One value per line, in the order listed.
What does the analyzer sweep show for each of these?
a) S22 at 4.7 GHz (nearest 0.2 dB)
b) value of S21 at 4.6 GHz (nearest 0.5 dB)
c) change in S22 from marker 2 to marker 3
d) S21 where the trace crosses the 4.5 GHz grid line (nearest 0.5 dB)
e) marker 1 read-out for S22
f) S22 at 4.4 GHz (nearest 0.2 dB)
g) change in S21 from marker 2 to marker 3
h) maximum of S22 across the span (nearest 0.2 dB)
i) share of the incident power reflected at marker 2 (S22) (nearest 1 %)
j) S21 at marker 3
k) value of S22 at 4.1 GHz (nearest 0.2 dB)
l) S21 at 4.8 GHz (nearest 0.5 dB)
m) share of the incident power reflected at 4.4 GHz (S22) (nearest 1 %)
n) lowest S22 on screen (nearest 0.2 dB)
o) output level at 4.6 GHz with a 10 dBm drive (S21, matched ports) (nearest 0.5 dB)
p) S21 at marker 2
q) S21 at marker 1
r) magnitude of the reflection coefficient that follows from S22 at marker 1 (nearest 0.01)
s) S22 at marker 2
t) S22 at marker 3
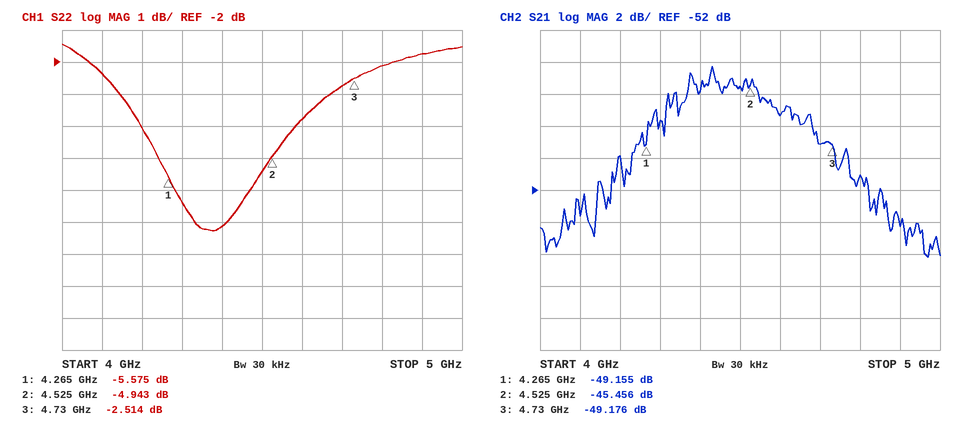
-2.8 dB
-47.5 dB
2.429 dB
-45.5 dB
-5.575 dB
-7.2 dB
-3.720 dB
-1.4 dB
32 %
-49.176 dB
-2.4 dB
-51.0 dB
19 %
-7.2 dB
-37.5 dBm
-45.456 dB
-49.155 dB
0.53
-4.943 dB
-2.514 dB
